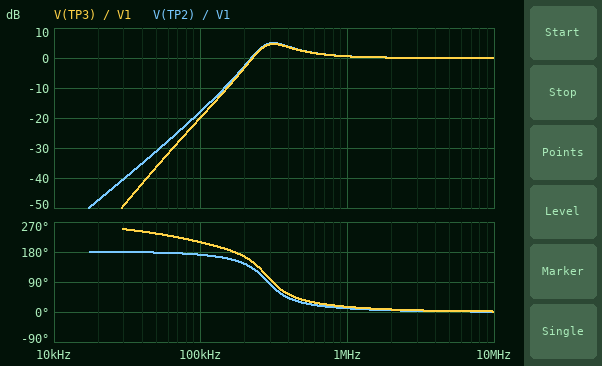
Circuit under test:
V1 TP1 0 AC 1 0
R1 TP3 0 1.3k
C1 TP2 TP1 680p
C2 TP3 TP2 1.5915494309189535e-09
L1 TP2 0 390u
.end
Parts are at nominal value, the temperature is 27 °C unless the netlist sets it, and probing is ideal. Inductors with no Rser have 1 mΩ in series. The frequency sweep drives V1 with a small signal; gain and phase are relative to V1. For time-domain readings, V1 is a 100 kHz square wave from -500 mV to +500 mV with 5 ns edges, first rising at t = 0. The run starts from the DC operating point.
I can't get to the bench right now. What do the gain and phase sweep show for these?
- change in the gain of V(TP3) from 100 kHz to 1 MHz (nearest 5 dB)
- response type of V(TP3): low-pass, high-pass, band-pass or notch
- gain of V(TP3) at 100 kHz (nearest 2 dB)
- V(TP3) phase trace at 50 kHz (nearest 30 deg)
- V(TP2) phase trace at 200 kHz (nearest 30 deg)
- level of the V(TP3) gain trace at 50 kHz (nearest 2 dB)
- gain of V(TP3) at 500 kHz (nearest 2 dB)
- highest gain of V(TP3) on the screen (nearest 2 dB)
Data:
20 dB
high-pass
-20 dB
240 deg
150 deg
-36 dB
2 dB
4 dB
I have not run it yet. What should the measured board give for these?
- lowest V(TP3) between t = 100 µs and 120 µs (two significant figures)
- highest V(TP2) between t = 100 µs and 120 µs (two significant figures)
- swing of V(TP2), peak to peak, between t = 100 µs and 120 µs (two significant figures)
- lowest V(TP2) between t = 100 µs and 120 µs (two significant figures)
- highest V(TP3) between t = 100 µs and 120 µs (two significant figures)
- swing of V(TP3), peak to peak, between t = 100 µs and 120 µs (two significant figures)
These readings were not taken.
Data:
-1.1 V
1.1 V
2.1 V
-1.1 V
1.1 V
2.1 V
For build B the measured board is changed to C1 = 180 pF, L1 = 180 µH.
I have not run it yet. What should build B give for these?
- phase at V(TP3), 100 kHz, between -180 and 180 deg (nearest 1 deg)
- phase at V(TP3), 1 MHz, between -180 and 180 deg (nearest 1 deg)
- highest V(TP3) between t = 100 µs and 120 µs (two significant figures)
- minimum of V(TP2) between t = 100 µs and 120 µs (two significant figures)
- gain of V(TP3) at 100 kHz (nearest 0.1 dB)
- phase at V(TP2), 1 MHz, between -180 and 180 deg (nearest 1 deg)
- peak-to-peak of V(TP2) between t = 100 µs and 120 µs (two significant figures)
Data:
-146 deg
73 deg
990 mV
-990 mV
-39.4 dB
68 deg
2.0 V
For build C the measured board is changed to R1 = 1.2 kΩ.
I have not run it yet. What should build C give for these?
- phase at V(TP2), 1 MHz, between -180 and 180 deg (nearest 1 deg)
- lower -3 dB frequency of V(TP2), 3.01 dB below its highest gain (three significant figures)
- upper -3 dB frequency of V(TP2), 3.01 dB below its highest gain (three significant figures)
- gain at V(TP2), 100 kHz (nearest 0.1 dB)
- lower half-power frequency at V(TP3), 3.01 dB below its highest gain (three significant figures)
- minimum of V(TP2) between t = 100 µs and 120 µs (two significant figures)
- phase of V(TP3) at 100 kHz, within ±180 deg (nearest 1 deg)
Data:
12 deg
236 kHz
644 kHz
-17.7 dB
239 kHz
-1.0 V
-149 deg
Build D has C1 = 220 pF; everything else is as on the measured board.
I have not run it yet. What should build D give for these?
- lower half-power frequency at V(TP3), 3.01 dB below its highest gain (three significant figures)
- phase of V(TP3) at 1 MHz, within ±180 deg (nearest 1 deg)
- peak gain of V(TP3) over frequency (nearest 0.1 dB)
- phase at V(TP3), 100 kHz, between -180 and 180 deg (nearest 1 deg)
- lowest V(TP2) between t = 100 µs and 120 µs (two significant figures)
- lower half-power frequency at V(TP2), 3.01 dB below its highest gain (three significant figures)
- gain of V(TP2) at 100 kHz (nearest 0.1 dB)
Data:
436 kHz
41 deg
0.7 dB
-150 deg
-990 mV
433 kHz
-28.3 dB
